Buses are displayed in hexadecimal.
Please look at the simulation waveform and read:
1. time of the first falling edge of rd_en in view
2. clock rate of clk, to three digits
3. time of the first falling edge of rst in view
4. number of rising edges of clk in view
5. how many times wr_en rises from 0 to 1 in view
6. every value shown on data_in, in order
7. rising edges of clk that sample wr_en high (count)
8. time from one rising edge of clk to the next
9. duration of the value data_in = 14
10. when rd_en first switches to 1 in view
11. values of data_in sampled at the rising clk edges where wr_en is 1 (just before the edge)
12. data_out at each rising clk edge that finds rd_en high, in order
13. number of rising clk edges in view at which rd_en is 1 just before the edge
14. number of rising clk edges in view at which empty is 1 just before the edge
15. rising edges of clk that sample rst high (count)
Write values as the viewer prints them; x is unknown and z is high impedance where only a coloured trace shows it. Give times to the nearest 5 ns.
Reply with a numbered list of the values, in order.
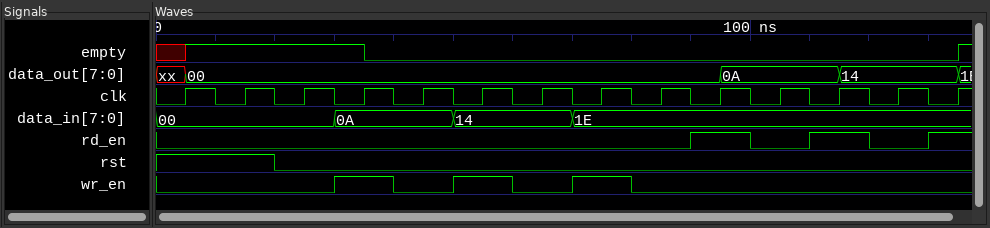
1. 100 ns
2. 100 MHz
3. 20 ns
4. 14
5. 3
6. 00, 0A, 14, 1E
7. 3
8. 10 ns
9. 20 ns
10. 90 ns
11. 0A, 14, 1E
12. 00, 0A, 14
13. 3
14. 3
15. 2
